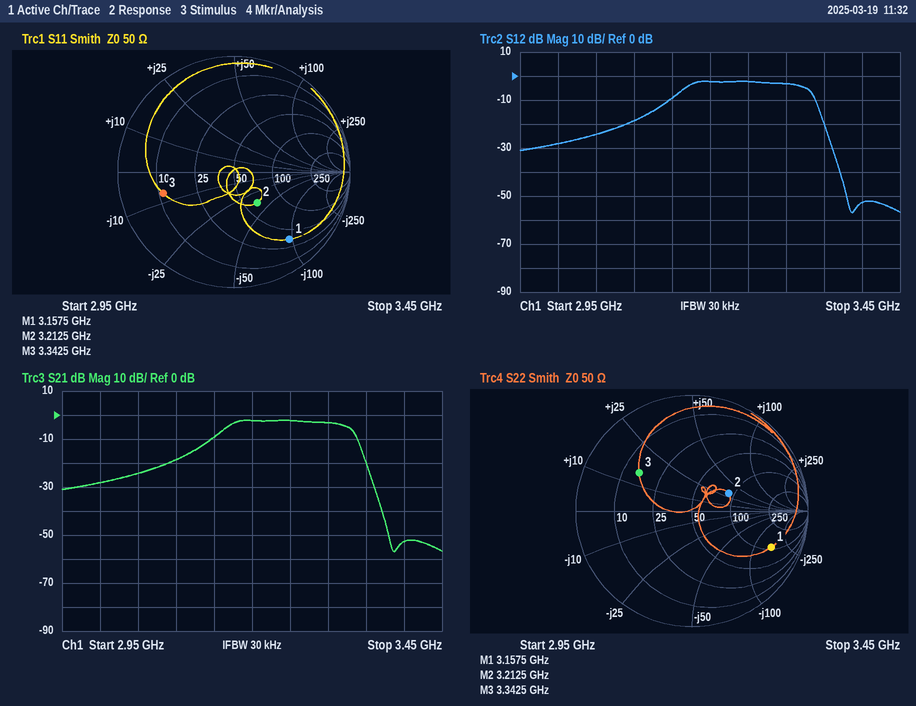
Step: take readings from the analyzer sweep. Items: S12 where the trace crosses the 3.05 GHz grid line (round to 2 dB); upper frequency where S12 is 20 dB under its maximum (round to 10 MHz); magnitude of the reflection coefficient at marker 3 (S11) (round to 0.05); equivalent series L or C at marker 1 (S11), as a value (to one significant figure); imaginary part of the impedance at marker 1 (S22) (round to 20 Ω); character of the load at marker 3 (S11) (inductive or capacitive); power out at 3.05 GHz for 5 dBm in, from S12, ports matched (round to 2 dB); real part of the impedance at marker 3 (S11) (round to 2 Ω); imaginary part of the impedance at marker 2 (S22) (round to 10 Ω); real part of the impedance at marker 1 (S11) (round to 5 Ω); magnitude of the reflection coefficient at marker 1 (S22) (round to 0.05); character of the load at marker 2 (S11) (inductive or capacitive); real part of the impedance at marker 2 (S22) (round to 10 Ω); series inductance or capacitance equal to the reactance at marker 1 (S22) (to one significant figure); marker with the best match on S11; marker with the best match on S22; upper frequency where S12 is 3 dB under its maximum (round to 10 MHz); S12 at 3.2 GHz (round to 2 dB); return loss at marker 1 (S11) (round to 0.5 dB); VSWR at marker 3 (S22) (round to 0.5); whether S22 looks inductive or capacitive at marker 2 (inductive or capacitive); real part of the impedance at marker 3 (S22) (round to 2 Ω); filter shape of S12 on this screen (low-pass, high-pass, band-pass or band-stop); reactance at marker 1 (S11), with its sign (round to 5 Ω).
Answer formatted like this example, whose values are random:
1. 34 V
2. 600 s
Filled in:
1. -24 dB
2. 3.35 GHz
3. 0.65
4. 500 fF
5. -160 Ω
6. capacitive
7. -20 dBm
8. 12 Ω
9. +30 Ω
10. 35 Ω
11. 0.75
12. capacitive
13. 90 Ω
14. 300 fF
15. marker 2
16. marker 2
17. 3.33 GHz
18. -2 dB
19. 2.5 dB
20. 3.5
21. inductive
22. 16 Ω
23. band-pass
24. -95 Ω
